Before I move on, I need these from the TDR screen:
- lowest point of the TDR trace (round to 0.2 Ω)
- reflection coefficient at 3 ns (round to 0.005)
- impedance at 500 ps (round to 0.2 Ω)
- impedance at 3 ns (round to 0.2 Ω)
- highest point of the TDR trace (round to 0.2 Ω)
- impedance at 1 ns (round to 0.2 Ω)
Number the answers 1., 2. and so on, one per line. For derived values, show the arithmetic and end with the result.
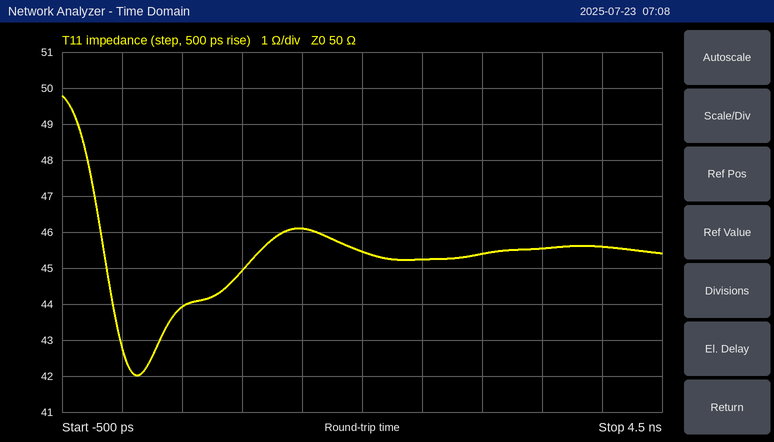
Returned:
1. 42.0 Ω
2. (45.4 − 50)/(45.4 + 50) ≈ -0.0482, so -0.050 to the nearest 0.005
3. 44.0 Ω
4. 45.4 Ω
5. 49.8 Ω
6. 45.0 Ω
